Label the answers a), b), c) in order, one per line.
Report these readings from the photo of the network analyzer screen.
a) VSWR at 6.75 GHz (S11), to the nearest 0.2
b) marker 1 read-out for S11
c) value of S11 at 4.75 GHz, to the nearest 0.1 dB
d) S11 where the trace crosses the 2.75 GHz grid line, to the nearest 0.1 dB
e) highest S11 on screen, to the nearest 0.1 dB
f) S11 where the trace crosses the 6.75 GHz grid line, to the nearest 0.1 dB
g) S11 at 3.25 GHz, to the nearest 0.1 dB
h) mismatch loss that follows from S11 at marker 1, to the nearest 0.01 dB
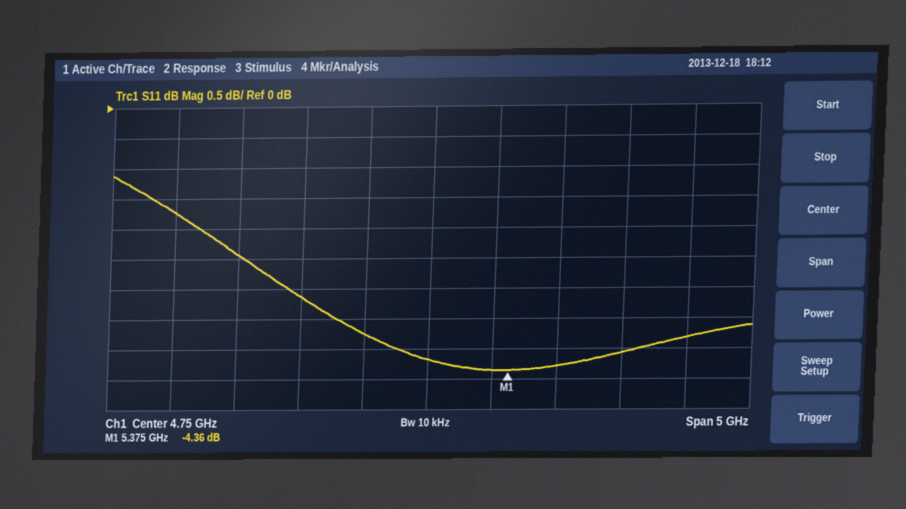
a) 4.6
b) -4.36 dB
c) -4.2 dB
d) -1.7 dB
e) -1.1 dB
f) -3.8 dB
g) -2.4 dB
h) 1.98 dB
